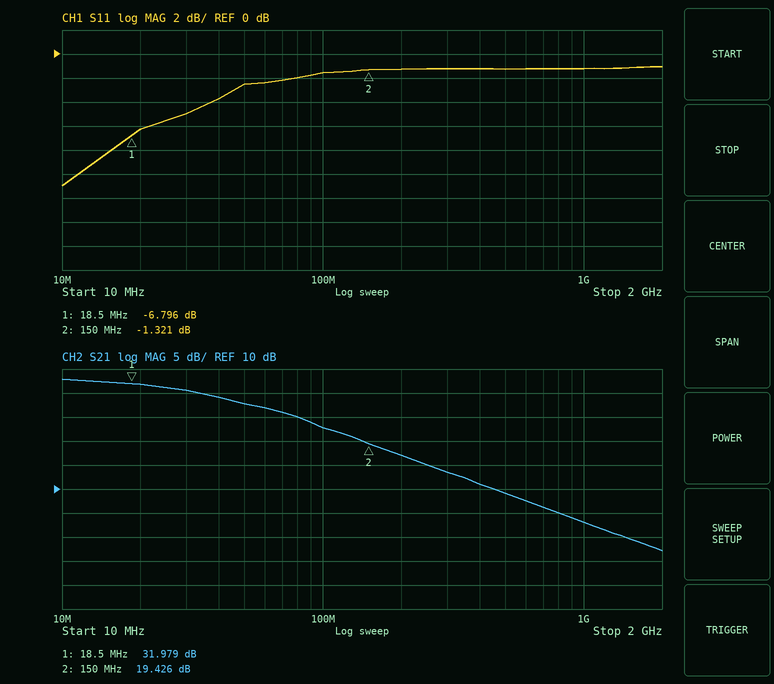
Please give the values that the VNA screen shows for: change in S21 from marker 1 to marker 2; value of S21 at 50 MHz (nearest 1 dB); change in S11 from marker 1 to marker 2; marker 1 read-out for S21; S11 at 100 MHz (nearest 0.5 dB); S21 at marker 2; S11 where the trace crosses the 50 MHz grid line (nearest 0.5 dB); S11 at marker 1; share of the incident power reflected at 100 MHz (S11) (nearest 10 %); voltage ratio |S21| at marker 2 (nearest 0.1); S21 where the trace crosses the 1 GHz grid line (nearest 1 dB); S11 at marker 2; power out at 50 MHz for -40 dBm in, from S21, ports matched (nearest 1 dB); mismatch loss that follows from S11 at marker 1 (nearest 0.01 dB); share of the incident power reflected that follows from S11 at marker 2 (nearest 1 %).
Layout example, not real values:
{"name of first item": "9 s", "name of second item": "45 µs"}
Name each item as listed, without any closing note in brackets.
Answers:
{"change in S21 from marker 1 to marker 2": "-12.553 dB", "value of S21 at 50 MHz": "28 dB", "change in S11 from marker 1 to marker 2": "5.475 dB", "marker 1 read-out for S21": "31.979 dB", "S11 at 100 MHz": "-1.5 dB", "S21 at marker 2": "19.426 dB", "S11 where the trace crosses the 50 MHz grid line": "-2.5 dB", "S11 at marker 1": "-6.796 dB", "share of the incident power reflected at 100 MHz (S11)": "70 %", "voltage ratio |S21| at marker 2": "9.4", "S21 where the trace crosses the 1 GHz grid line": "3 dB", "S11 at marker 2": "-1.321 dB", "power out at 50 MHz for -40 dBm in, from S21, ports matched": "-12 dBm", "mismatch loss that follows from S11 at marker 1": "1.02 dB", "share of the incident power reflected that follows from S11 at marker 2": "74 %"}
